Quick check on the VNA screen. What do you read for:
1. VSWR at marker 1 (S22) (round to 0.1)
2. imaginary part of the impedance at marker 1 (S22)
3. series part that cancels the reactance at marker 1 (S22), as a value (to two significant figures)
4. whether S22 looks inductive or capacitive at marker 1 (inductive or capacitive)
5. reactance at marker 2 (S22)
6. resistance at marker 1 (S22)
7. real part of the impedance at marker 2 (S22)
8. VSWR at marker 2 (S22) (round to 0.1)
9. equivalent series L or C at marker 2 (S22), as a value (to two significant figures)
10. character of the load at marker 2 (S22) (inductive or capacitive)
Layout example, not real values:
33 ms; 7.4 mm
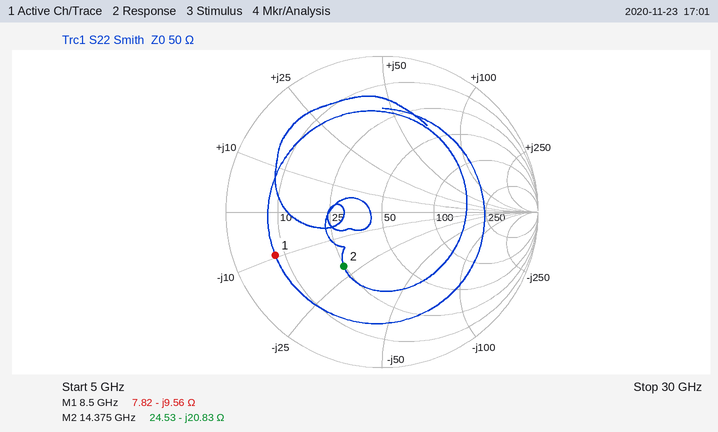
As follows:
6.6; -9.56 Ω; 180 pH; capacitive; -20.83 Ω; 7.82 Ω; 24.53 Ω; 2.5; 530 fF; capacitive
